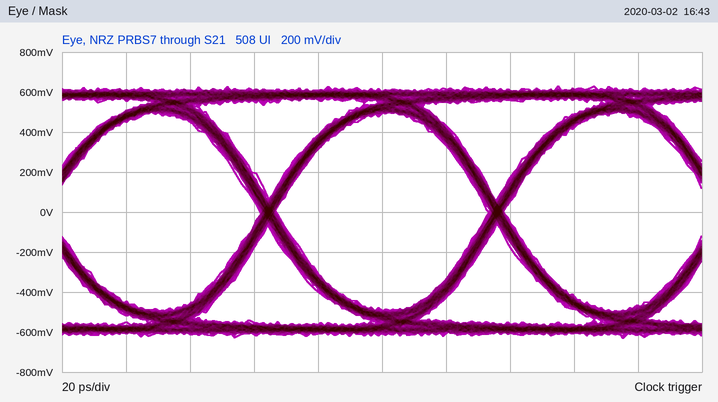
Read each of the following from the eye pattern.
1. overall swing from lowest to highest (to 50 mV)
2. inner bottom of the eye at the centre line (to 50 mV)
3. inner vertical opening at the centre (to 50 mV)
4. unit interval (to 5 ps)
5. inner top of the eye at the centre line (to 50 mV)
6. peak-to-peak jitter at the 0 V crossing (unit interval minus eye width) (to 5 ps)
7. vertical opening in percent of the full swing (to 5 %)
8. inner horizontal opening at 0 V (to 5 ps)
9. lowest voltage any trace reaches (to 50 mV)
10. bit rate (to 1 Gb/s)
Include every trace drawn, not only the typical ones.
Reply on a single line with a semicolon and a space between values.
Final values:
1.25 V; -500 mV; 1.00 V; 70 ps; 500 mV; 5 ps; 80 %; 65 ps; -650 mV; 14 Gb/s
